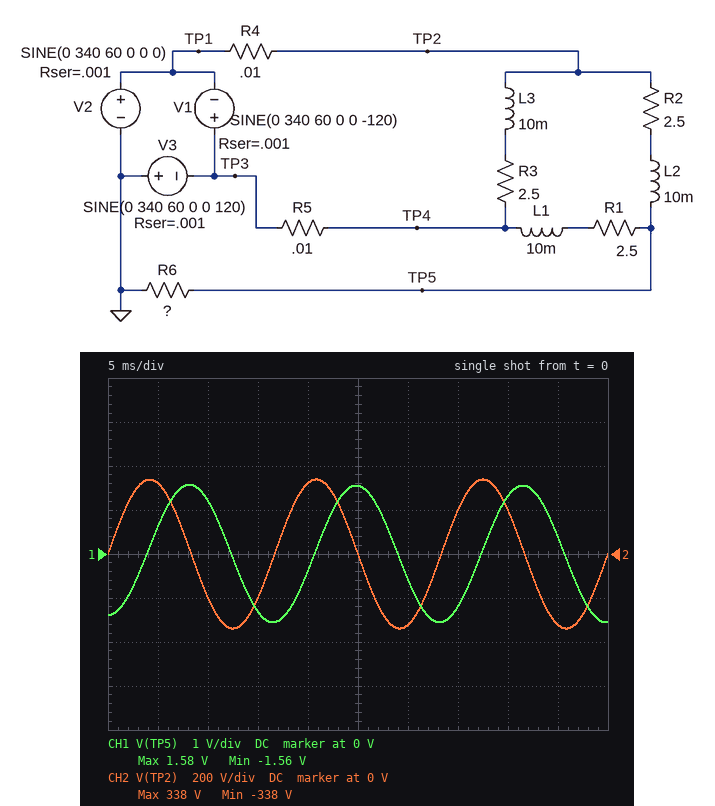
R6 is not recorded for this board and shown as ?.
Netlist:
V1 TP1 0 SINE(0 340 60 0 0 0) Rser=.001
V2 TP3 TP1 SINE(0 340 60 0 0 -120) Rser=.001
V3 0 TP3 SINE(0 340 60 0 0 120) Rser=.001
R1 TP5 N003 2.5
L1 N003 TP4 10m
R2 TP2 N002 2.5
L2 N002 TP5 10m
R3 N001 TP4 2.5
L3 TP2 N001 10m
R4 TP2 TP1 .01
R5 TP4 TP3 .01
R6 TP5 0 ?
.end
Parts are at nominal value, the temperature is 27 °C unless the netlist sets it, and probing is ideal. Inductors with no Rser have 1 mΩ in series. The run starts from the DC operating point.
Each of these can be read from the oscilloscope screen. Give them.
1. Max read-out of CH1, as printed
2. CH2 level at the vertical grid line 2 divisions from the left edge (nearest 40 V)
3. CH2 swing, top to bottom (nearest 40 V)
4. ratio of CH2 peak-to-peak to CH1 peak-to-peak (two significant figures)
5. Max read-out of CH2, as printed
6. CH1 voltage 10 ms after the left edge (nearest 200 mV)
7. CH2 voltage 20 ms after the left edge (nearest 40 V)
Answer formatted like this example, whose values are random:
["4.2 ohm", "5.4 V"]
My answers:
["1.58 V", "-200 V", "680 V", "220", "338 V", "1.2 V", "320 V"]
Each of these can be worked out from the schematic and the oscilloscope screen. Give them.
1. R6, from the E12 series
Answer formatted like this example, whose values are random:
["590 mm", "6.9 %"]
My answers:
["0.012 Ω"]
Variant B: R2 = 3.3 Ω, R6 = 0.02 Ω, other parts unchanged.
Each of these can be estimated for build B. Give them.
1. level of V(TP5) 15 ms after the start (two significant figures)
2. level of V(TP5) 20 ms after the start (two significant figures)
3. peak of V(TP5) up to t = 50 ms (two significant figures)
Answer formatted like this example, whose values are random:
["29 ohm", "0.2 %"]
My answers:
["-2.1 V", "-500 mV", "2.4 V"]
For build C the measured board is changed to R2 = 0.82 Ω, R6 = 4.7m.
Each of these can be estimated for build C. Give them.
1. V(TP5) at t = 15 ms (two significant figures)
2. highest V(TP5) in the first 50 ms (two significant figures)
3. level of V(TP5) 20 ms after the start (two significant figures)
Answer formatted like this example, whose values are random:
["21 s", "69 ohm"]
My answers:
["-440 mV", "890 mV", "-210 mV"]
